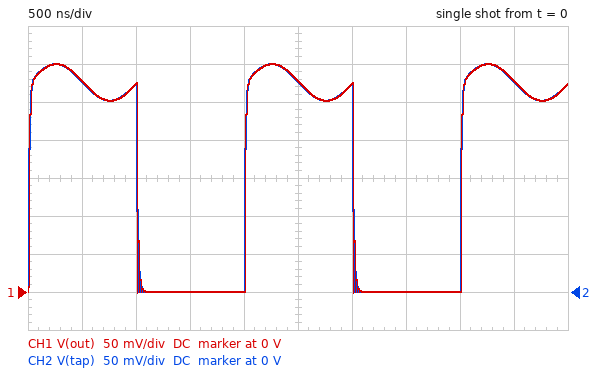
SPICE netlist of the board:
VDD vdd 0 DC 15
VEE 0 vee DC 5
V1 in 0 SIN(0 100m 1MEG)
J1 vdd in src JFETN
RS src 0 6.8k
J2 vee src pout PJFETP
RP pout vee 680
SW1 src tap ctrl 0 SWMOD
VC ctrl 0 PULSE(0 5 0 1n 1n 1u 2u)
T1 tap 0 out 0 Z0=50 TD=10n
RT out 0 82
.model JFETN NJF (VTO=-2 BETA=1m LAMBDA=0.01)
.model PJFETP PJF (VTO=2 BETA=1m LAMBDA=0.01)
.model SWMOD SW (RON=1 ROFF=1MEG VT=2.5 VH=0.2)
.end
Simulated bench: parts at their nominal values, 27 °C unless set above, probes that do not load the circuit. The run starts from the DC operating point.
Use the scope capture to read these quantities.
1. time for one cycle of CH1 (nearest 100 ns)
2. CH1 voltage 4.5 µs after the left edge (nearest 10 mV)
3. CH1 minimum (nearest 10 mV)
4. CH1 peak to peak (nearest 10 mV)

2.0 µs
280 mV
0 V
300 mV
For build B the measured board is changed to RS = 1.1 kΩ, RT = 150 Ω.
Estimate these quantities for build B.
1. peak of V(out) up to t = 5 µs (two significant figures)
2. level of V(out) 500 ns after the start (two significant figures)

420 mV
390 mV
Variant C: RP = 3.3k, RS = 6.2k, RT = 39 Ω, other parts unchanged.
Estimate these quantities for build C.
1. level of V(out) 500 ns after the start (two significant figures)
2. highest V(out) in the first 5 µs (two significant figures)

150 mV
170 mV
